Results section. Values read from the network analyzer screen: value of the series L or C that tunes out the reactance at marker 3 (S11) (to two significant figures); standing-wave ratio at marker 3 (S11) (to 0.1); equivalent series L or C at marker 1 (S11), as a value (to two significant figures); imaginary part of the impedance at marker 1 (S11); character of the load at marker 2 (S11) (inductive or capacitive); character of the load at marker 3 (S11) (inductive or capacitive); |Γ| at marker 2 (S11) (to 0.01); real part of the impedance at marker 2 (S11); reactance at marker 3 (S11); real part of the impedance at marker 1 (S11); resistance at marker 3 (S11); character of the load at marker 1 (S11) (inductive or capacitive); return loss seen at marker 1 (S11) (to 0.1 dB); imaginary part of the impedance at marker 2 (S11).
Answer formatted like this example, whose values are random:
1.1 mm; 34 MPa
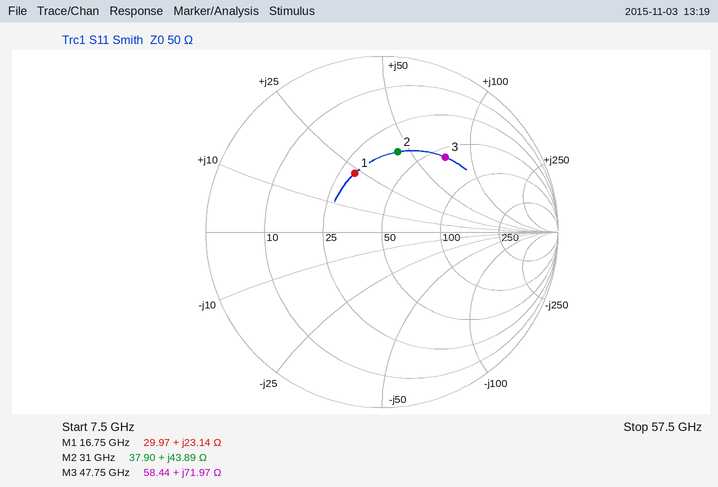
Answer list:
46 fF; 3.5; 220 pH; +23.14 Ω; inductive; inductive; 0.46; 37.90 Ω; +71.97 Ω; 29.97 Ω; 58.44 Ω; inductive; 8.7 dB; +43.89 Ω
